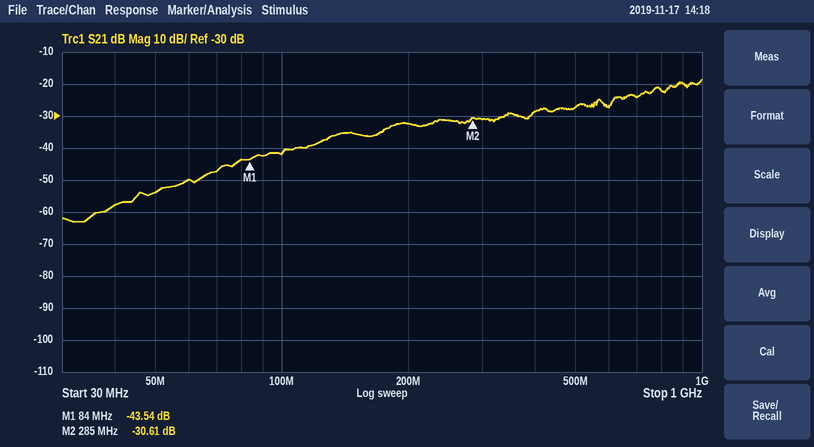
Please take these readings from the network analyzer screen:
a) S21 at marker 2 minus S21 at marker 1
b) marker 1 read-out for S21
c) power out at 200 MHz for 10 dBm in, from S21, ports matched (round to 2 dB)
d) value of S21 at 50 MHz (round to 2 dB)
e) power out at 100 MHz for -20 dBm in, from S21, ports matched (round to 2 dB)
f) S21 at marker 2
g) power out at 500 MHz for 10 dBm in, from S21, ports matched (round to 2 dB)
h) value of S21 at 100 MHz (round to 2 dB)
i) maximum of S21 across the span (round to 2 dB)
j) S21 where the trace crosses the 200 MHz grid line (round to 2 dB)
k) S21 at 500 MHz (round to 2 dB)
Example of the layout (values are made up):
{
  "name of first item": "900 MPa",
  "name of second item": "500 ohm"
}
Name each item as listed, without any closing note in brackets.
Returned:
{
  "S21 at marker 2 minus S21 at marker 1": "12.93 dB",
  "marker 1 read-out for S21": "-43.54 dB",
  "power out at 200 MHz for 10 dBm in, from S21, ports matched": "-22 dBm",
  "value of S21 at 50 MHz": "-54 dB",
  "power out at 100 MHz for -20 dBm in, from S21, ports matched": "-62 dBm",
  "S21 at marker 2": "-30.61 dB",
  "power out at 500 MHz for 10 dBm in, from S21, ports matched": "-18 dBm",
  "value of S21 at 100 MHz": "-42 dB",
  "maximum of S21 across the span": "-18 dB",
  "S21 where the trace crosses the 200 MHz grid line": "-32 dB",
  "S21 at 500 MHz": "-28 dB"
}
